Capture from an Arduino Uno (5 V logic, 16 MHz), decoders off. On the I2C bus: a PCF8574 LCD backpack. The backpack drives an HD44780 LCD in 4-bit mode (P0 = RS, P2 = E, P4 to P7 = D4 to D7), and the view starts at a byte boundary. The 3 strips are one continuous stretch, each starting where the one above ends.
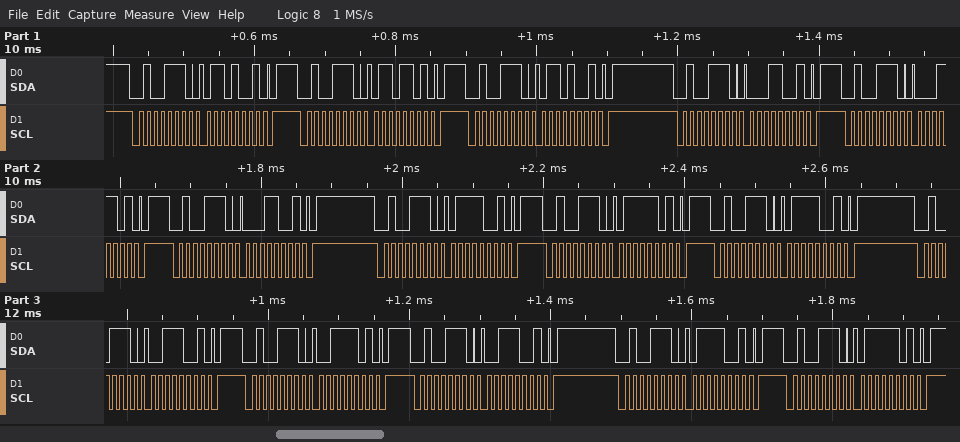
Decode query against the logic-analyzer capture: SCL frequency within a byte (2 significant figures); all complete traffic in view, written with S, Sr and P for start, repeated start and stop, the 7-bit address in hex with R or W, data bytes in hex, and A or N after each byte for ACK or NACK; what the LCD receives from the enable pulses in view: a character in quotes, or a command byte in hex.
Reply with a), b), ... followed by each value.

a) 100 kHz
b) S 27W A 69 A P S 27W A 6D A P S 27W A 69 A P S 27W A 19 A P S 27W A 1D A P S 27W A 19 A P S 27W A 79 A P S 27W A 7D A P S 27W A 79 A P S 27W A 39 A P S 27W A 3D A P S 27W A 39 A P S 27W A 79 A P S 27W A 7D A P
c) 'a' 's'
